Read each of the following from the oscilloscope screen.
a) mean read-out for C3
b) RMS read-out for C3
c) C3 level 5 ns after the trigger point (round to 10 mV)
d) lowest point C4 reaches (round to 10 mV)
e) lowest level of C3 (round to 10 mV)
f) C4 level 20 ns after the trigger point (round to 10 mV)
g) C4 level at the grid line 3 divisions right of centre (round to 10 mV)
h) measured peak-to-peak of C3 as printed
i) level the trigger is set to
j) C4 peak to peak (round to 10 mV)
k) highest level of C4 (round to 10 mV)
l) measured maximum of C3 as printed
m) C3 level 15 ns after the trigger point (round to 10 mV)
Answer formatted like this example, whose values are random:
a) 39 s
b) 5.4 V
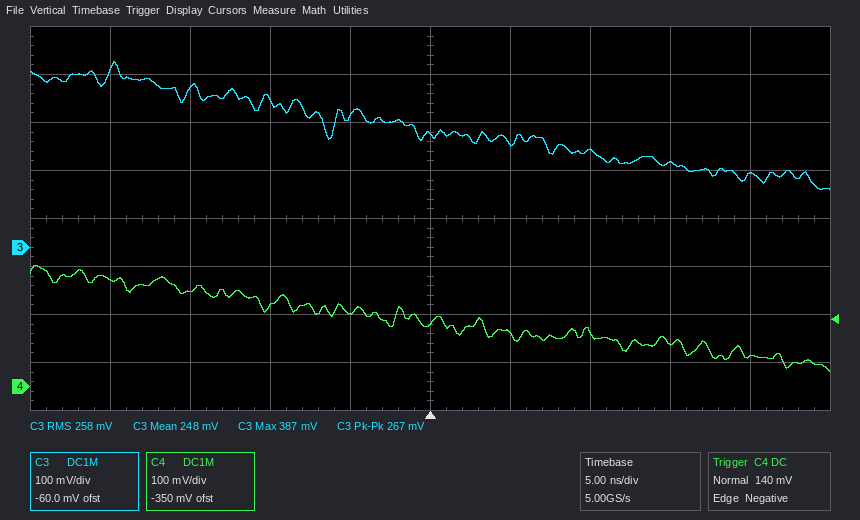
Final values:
a) 248 mV
b) 258 mV
c) 220 mV
d) 30 mV
e) 120 mV
f) 60 mV
g) 90 mV
h) 267 mV
i) 140 mV
j) 220 mV
k) 250 mV
l) 387 mV
m) 180 mV
